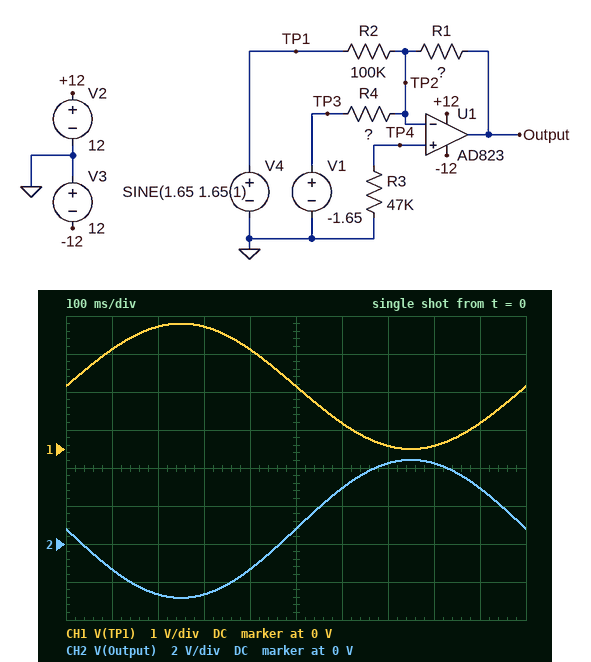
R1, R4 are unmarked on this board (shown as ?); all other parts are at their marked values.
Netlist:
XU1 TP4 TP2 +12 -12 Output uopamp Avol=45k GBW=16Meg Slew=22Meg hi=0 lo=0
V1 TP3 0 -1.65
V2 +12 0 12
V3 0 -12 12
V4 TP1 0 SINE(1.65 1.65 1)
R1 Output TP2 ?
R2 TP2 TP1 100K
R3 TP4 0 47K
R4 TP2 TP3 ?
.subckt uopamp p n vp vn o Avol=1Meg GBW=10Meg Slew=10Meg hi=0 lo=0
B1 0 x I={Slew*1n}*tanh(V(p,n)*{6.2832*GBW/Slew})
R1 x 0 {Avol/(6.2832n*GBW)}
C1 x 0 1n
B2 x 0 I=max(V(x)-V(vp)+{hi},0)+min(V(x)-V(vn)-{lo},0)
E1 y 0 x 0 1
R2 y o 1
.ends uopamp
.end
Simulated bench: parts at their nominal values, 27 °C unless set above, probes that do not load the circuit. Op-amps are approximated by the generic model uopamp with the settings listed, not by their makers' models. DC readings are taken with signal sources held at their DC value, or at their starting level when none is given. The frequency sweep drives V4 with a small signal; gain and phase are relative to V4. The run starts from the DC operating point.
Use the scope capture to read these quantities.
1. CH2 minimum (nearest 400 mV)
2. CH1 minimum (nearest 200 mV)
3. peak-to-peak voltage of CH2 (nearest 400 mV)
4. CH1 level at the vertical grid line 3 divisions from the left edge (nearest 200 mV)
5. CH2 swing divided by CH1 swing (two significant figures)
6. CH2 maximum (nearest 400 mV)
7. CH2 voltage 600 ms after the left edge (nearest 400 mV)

-2.8 V
0 V
7.2 V
3.2 V
2.2
4.4 V
2.8 V
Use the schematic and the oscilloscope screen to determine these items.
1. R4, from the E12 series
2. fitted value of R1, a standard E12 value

82 kΩ
220 kΩ
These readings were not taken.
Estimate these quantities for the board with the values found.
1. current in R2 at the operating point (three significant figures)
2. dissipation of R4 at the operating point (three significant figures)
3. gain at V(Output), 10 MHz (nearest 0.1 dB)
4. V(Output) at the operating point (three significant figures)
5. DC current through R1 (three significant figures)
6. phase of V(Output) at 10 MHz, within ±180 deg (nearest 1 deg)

16.5 µA
33.2 µW
-4.8 dB
797 mV
3.62 µA
105 deg
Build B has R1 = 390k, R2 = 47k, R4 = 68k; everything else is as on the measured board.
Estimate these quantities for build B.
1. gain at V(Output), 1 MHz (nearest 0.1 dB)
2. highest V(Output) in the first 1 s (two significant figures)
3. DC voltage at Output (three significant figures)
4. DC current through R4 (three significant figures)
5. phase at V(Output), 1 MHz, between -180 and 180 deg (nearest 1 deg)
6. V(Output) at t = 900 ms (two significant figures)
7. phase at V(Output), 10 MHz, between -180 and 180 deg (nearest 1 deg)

15.6 dB
9.5 V
-4.23 V
24.3 µA
137 deg
3.8 V
96 deg
